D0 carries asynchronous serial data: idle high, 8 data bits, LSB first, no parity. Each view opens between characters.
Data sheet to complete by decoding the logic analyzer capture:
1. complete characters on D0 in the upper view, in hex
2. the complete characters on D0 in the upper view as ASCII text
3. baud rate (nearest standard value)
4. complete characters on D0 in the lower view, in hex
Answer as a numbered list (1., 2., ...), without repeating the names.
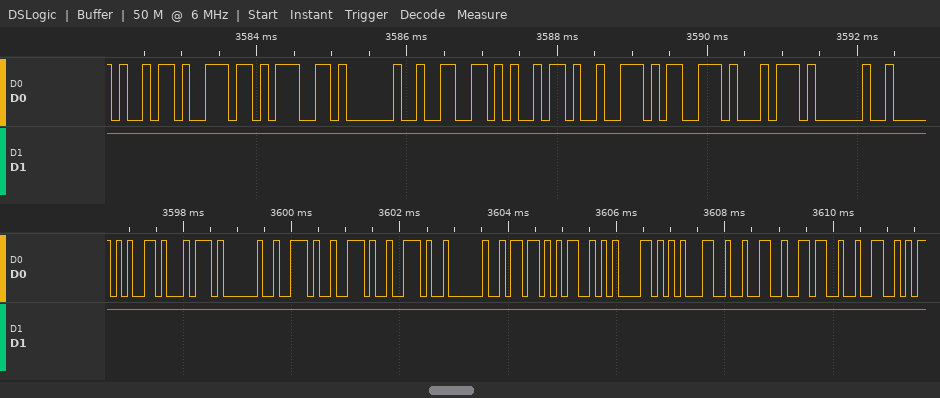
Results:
1. 69, 6E, 67, 20, 66, 69, 72, 73, 74, 20
2. "ing first "
3. 9600 baud
4. 65, 74, 20, 2E, 2E, 2E, 20, 5B, 53, 58, 31, 32, 36, 32
